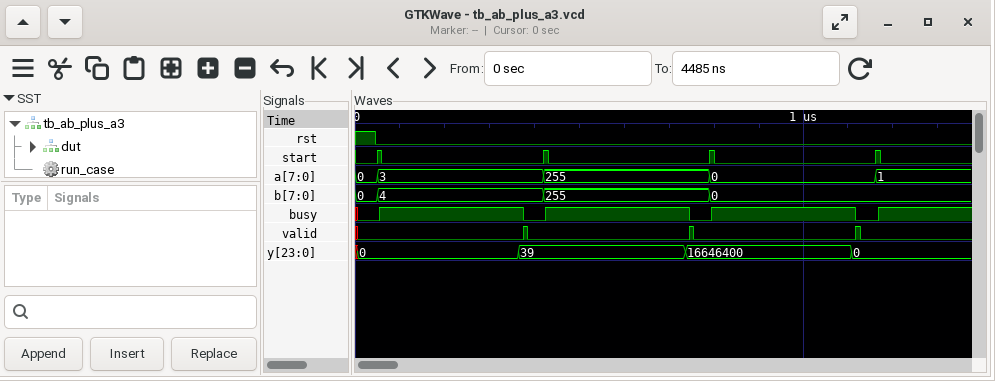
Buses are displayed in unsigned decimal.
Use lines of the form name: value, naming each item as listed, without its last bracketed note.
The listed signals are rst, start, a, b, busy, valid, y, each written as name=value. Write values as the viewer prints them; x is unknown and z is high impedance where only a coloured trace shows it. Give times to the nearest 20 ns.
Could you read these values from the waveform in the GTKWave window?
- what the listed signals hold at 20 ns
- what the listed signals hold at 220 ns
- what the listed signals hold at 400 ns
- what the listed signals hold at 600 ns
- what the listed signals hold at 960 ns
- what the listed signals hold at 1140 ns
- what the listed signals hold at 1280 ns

what the listed signals hold at 20 ns: rst=1, start=0, a=0, b=0, busy=0, valid=0, y=0
what the listed signals hold at 220 ns: rst=0, start=0, a=3, b=4, busy=1, valid=0, y=0
what the listed signals hold at 400 ns: rst=0, start=0, a=3, b=4, busy=0, valid=0, y=39
what the listed signals hold at 600 ns: rst=0, start=0, a=255, b=255, busy=1, valid=0, y=39
what the listed signals hold at 960 ns: rst=0, start=0, a=0, b=0, busy=1, valid=0, y=16646400
what the listed signals hold at 1140 ns: rst=0, start=0, a=0, b=0, busy=0, valid=0, y=0
what the listed signals hold at 1280 ns: rst=0, start=0, a=1, b=0, busy=1, valid=0, y=0
